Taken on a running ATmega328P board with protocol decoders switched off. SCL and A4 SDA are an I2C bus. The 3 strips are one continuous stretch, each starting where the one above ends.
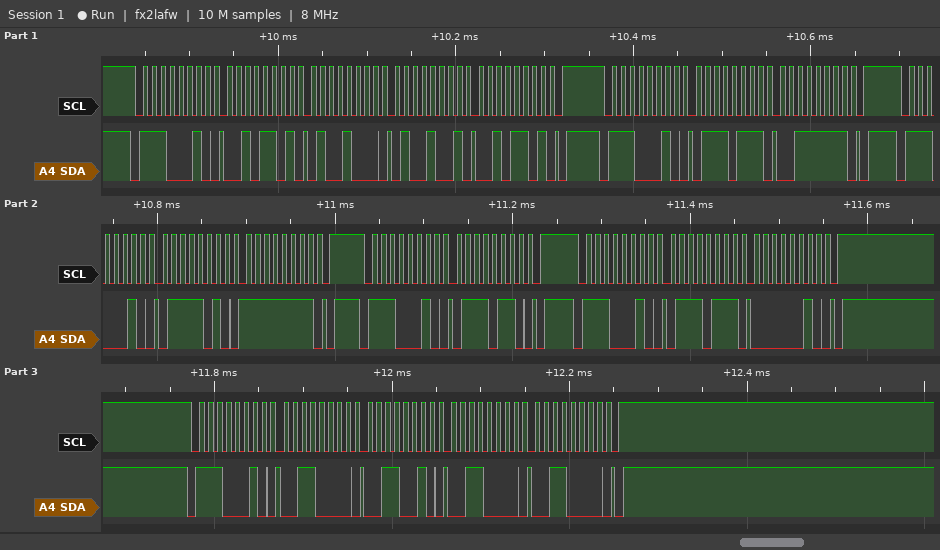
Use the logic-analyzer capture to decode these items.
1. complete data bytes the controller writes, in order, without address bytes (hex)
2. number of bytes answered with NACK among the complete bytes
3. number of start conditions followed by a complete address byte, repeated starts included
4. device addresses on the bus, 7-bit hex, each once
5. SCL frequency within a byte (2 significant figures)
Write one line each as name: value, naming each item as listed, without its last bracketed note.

complete data bytes the controller writes, in order, without address bytes: 2D 48 49 2D 77 3F 7A FF 76 77 02 30 32 30 30
number of bytes answered with NACK among the complete bytes: 0
number of start conditions followed by a complete address byte, repeated starts included: 6
device addresses on the bus, 7-bit hex, each once: 0x71
SCL frequency within a byte: 100 kHz
